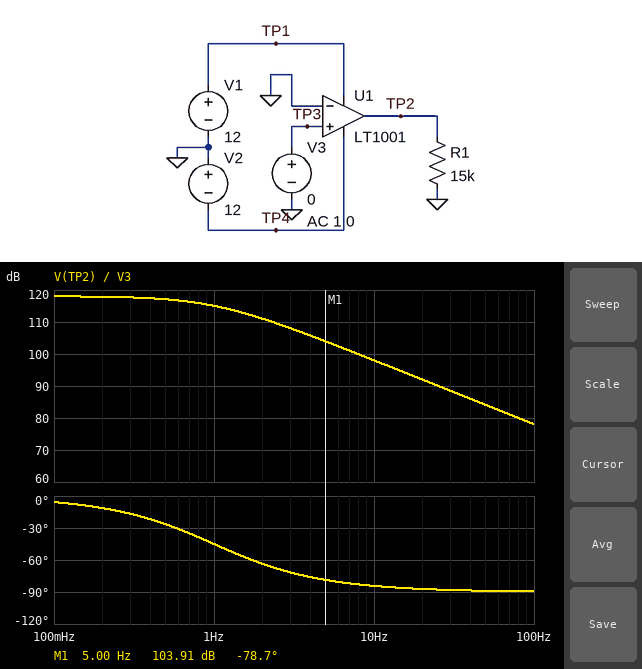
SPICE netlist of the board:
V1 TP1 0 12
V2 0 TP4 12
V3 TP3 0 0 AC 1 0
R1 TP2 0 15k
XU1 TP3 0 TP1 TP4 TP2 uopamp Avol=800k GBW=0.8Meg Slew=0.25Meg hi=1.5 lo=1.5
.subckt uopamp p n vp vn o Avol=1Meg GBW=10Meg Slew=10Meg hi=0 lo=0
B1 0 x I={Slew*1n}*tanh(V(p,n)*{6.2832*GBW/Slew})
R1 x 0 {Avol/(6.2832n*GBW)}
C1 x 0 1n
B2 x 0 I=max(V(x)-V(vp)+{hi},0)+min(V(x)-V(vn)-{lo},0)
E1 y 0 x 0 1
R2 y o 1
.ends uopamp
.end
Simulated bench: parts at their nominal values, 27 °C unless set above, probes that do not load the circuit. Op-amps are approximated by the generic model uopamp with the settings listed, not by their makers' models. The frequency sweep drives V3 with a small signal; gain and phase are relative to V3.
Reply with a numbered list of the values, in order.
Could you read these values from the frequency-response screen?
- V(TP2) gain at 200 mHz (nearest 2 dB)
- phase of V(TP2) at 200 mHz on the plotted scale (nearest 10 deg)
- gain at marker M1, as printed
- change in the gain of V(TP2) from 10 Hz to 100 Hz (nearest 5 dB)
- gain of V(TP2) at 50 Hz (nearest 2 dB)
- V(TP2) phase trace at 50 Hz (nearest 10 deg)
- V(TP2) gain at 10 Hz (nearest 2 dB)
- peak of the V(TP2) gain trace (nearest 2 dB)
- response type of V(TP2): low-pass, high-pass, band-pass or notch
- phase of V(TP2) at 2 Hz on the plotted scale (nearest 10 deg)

1. 118 dB
2. -10 deg
3. 103.91 dB
4. -20 dB
5. 84 dB
6. -90 deg
7. 98 dB
8. 118 dB
9. low-pass
10. -60 deg
